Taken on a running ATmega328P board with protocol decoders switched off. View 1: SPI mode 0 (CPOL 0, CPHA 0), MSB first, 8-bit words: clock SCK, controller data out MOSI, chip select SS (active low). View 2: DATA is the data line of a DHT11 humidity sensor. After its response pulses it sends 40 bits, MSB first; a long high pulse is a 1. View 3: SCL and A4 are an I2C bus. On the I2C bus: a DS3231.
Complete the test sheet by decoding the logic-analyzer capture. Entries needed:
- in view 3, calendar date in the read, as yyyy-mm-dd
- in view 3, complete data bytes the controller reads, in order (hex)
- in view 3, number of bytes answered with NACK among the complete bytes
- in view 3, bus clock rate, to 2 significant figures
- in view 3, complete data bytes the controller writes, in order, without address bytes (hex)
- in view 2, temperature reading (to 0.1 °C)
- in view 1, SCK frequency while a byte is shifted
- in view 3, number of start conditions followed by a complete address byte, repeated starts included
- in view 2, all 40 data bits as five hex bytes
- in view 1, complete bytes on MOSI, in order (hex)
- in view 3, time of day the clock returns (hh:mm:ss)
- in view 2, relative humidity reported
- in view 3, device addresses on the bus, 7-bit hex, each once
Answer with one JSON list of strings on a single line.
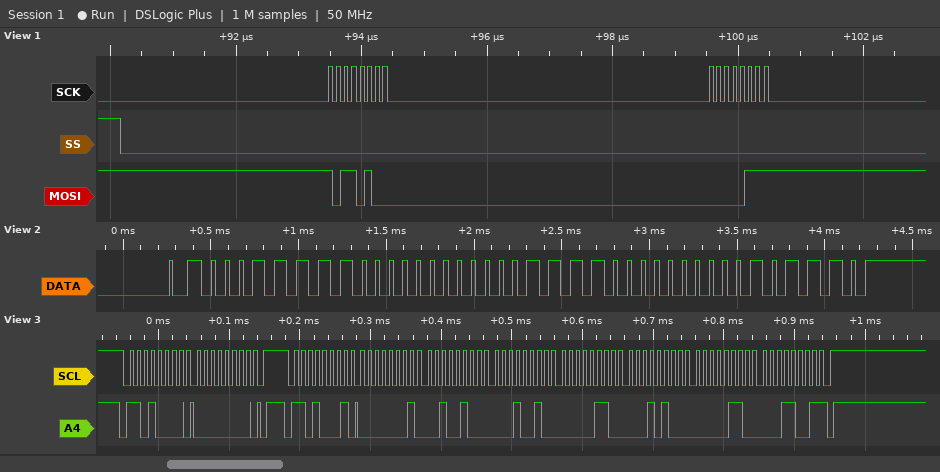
["2019-06-14", "01 24 12 06 14 06 19", "1", "100 kHz", "00", "15.0 °C", "8 MHz", "2", "1F 00 0F 00 2E", "B4 07", "12:24:01", "31 %", "0x68"]
